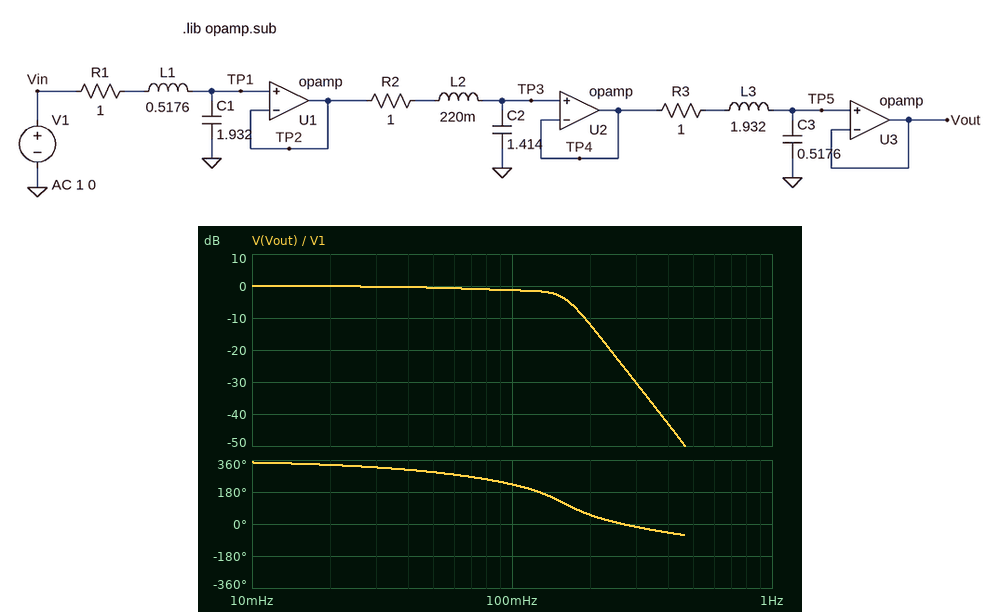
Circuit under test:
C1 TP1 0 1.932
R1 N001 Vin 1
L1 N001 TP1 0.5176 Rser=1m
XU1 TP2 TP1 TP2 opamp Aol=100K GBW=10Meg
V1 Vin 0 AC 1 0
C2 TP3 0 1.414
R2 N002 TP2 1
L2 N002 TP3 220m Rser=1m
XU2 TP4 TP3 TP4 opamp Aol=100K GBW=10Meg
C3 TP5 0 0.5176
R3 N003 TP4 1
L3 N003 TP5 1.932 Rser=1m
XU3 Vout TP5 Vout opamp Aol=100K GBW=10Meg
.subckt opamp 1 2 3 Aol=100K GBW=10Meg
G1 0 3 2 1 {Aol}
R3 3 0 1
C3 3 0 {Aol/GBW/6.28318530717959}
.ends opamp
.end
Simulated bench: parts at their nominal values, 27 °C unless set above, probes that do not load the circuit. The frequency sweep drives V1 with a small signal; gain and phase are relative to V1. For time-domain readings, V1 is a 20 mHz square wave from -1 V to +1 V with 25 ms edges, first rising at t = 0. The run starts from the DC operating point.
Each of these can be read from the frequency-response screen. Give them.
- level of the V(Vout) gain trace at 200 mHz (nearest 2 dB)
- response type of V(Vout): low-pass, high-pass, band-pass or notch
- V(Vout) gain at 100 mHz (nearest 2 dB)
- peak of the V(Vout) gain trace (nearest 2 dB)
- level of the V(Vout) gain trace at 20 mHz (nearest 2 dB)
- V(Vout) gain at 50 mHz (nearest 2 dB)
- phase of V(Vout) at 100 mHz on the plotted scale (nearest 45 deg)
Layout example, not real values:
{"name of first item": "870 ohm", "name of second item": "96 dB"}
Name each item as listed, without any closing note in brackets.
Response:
{"level of the V(Vout) gain trace at 200 mHz": "-12 dB", "response type of V(Vout): low-pass, high-pass, band-pass or notch": "low-pass", "V(Vout) gain at 100 mHz": "-2 dB", "peak of the V(Vout) gain trace": "0 dB", "level of the V(Vout) gain trace at 20 mHz": "0 dB", "V(Vout) gain at 50 mHz": "0 dB", "phase of V(Vout) at 100 mHz on the plotted scale": "225 deg"}
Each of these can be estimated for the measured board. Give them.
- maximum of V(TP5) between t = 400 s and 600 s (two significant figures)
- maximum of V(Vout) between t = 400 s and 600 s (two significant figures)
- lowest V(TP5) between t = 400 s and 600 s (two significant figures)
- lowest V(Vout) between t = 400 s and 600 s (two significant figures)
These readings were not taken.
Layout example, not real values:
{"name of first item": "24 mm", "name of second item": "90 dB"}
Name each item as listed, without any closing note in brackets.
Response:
{"maximum of V(TP5) between t = 400 s and 600 s": "1.1 V", "maximum of V(Vout) between t = 400 s and 600 s": "1.1 V", "lowest V(TP5) between t = 400 s and 600 s": "-1.1 V", "lowest V(Vout) between t = 400 s and 600 s": "-1.1 V"}
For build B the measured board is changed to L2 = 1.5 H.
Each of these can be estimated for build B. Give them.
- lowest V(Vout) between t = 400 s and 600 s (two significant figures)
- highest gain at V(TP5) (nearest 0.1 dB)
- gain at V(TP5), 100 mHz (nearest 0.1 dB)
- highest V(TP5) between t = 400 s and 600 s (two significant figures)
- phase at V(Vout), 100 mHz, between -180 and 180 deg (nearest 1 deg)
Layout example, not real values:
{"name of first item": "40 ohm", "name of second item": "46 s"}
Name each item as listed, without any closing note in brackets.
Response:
{"lowest V(Vout) between t = 400 s and 600 s": "-1.5 V", "highest gain at V(TP5)": "1.7 dB", "gain at V(TP5), 100 mHz": "1.5 dB", "highest V(TP5) between t = 400 s and 600 s": "1.5 V", "phase at V(Vout), 100 mHz, between -180 and 180 deg": "-171 deg"}
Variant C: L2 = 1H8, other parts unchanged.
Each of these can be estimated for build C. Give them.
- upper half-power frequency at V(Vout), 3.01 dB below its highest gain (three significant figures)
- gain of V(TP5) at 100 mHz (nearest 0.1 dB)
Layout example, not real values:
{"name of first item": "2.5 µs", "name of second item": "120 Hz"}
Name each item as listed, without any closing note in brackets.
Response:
{"upper half-power frequency at V(Vout), 3.01 dB below its highest gain": "125 mHz", "gain of V(TP5) at 100 mHz": "1.6 dB"}
